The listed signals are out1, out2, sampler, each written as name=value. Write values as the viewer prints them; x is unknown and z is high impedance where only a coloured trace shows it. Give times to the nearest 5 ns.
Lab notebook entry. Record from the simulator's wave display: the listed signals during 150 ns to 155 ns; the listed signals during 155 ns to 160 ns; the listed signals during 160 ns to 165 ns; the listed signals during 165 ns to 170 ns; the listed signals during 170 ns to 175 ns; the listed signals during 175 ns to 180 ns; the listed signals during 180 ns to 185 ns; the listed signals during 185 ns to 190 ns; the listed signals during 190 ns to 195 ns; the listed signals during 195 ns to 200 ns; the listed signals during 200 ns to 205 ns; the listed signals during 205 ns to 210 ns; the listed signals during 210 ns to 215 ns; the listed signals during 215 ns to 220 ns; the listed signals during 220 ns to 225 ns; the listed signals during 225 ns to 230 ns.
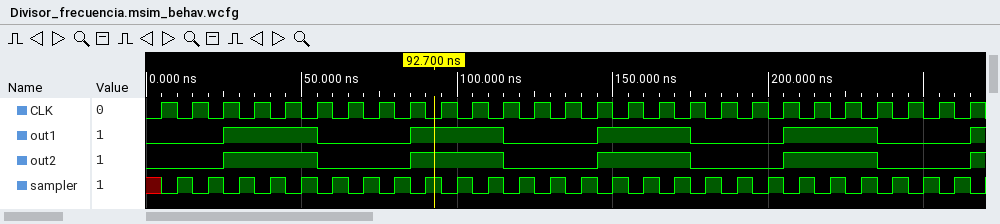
out1=1, out2=1, sampler=1
out1=1, out2=1, sampler=0
out1=1, out2=1, sampler=1
out1=1, out2=1, sampler=0
out1=1, out2=1, sampler=1
out1=0, out2=0, sampler=0
out1=0, out2=0, sampler=1
out1=0, out2=0, sampler=0
out1=0, out2=0, sampler=1
out1=0, out2=0, sampler=0
out1=0, out2=0, sampler=1
out1=1, out2=1, sampler=0
out1=1, out2=1, sampler=1
out1=1, out2=1, sampler=0
out1=1, out2=1, sampler=1
out1=1, out2=1, sampler=0
